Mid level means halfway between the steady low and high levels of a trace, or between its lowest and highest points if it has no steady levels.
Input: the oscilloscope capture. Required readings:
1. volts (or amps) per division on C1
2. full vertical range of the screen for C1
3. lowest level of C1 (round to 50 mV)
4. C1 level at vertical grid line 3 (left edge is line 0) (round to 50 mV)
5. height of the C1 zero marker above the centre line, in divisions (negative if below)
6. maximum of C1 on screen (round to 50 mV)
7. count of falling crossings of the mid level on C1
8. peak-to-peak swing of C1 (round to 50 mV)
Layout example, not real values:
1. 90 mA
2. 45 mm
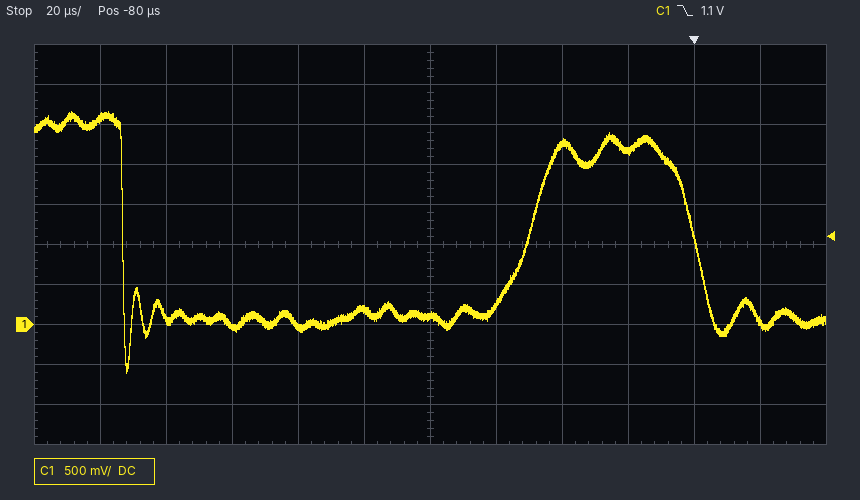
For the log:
1. 500 mV
2. 5 V
3. -600 mV
4. 0 mV
5. -2.0 div
6. 2.65 V
7. 2
8. 3.25 V
